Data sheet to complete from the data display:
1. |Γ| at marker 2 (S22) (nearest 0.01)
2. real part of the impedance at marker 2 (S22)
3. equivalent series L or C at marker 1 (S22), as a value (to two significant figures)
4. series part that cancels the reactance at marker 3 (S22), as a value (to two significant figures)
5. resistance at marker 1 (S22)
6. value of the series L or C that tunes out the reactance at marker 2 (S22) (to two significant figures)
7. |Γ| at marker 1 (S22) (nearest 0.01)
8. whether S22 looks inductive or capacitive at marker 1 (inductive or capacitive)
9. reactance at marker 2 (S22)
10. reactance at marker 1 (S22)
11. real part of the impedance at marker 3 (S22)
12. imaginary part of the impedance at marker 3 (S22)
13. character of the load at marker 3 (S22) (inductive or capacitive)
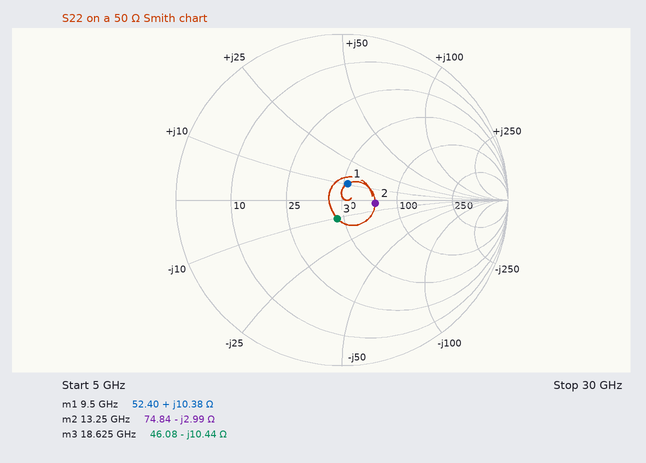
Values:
0.20
74.84 Ω
170 pH
89 pH
52.40 Ω
36 pH
0.10
inductive
-2.99 Ω
+10.38 Ω
46.08 Ω
-10.44 Ω
capacitive
